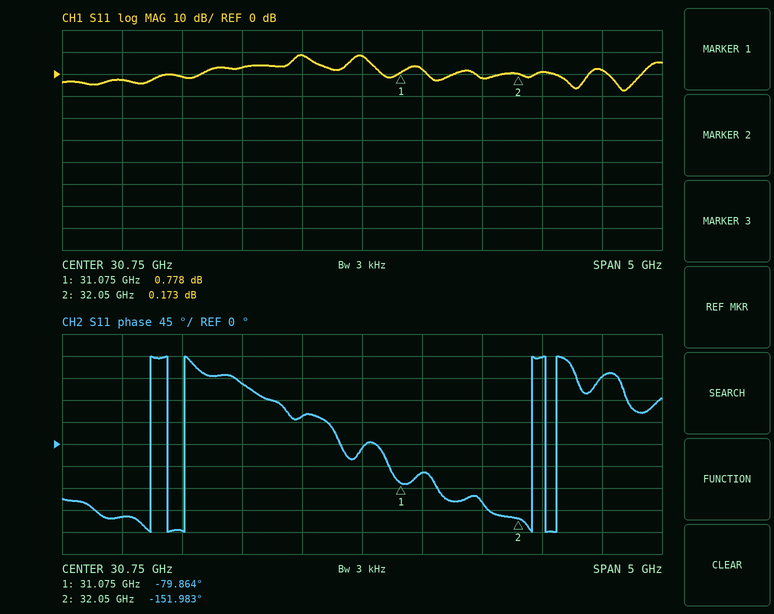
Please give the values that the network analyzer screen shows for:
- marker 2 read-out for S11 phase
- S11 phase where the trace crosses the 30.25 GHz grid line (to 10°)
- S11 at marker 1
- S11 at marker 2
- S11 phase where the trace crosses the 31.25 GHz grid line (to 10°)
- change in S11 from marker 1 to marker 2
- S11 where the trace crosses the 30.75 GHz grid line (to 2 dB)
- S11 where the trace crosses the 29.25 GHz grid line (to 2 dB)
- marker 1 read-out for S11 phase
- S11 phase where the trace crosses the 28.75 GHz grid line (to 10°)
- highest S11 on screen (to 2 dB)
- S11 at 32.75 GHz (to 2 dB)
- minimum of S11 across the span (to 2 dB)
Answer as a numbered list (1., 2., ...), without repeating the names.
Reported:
1. -151.983°
2. 60°
3. 0.778 dB
4. 0.173 dB
5. -60°
6. -0.605 dB
7. 8 dB
8. -2 dB
9. -79.864°
10. -150°
11. 8 dB
12. 2 dB
13. -8 dB
